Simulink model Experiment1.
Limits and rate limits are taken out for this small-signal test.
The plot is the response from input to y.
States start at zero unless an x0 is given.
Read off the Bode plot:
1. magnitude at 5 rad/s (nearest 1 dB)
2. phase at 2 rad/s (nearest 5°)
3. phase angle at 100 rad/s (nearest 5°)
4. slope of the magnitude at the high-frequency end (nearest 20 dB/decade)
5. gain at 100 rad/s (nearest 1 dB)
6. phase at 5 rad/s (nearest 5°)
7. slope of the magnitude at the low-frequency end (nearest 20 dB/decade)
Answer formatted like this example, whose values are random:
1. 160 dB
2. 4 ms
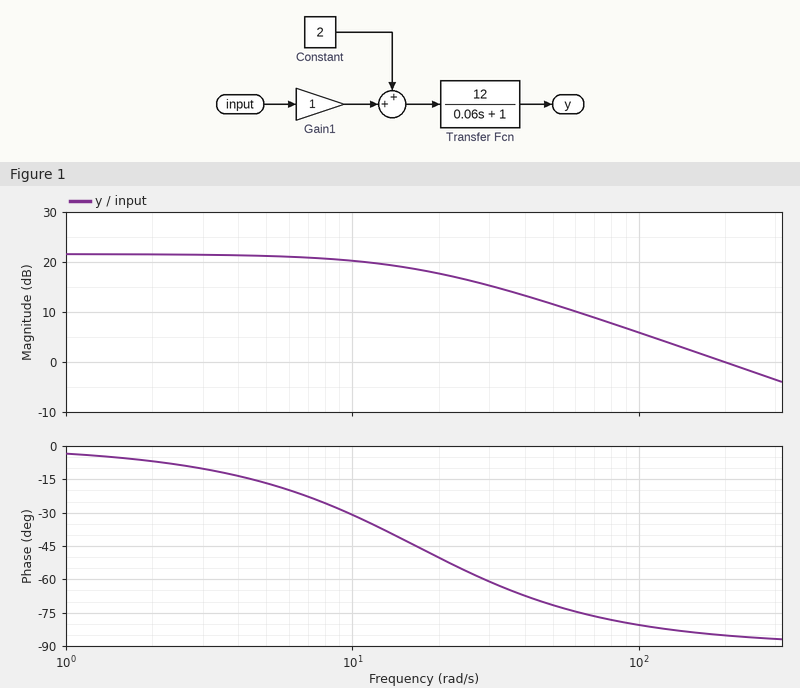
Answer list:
1. 21 dB
2. -5°
3. -80°
4. -20 dB/decade
5. 6 dB
6. -15°
7. 0 dB/decade
